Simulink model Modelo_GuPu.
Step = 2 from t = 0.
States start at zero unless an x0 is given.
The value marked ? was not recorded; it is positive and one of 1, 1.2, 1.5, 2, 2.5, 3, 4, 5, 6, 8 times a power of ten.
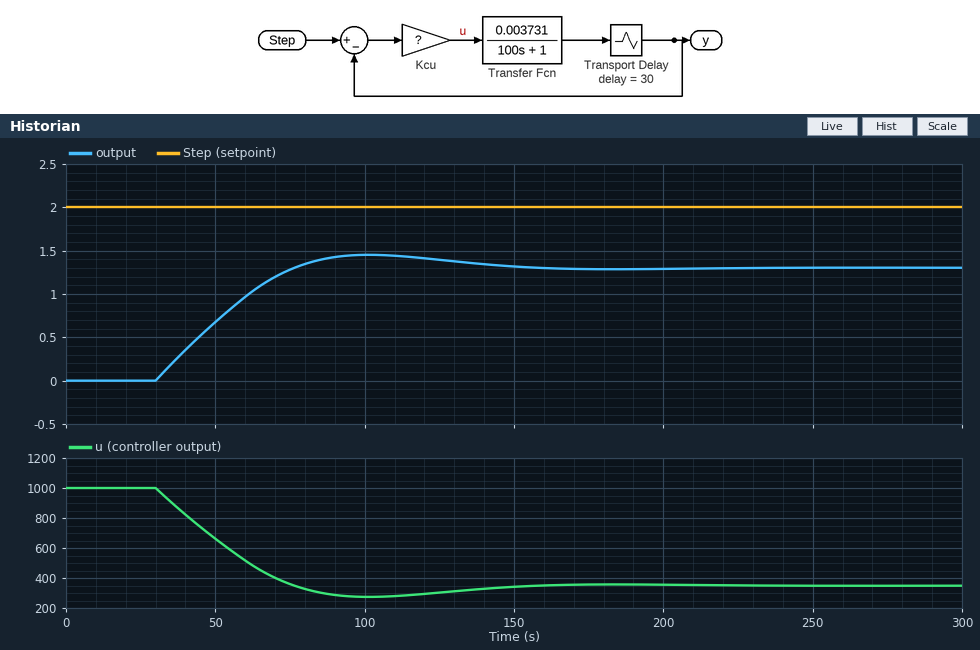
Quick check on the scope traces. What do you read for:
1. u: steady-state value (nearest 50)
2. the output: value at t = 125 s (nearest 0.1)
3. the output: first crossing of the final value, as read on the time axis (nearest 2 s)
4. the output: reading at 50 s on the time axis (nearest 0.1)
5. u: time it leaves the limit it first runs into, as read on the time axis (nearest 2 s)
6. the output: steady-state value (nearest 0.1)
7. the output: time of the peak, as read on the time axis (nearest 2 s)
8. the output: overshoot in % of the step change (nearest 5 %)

350
1.4
76 s
0.7
30 s
1.3
102 s
10 %
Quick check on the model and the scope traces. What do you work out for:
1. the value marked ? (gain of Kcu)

500
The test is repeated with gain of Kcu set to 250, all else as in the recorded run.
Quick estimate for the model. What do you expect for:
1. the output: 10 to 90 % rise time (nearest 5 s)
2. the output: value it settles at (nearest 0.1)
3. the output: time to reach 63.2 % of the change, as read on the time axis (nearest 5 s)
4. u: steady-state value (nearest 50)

75 s
1.0
70 s
250
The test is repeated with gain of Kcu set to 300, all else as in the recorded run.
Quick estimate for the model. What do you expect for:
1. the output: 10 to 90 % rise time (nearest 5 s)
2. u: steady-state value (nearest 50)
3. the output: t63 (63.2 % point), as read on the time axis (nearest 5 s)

60 s
300
65 s
